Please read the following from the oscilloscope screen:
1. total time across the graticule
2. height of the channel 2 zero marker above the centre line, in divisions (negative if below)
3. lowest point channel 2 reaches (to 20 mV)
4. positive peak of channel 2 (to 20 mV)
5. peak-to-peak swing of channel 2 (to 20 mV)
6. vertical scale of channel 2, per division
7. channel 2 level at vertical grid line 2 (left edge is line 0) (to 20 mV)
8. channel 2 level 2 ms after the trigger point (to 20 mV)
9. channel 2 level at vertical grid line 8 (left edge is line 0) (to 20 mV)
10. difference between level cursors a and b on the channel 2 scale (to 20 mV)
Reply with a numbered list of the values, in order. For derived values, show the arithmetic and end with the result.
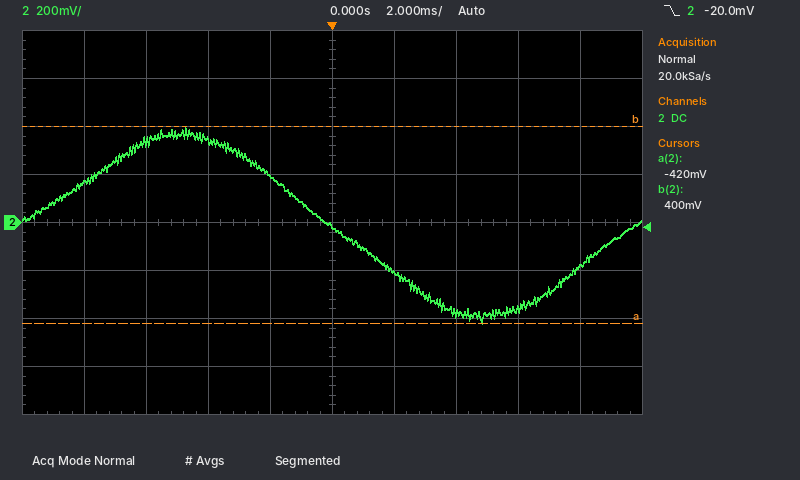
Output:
1. 20 ms
2. 0.0 div
3. -420 mV
4. 400 mV
5. 400 mV − (-420 mV) = 820 mV
6. 200 mV
7. 340 mV
8. -200 mV
9. -360 mV
10. 820 mV
